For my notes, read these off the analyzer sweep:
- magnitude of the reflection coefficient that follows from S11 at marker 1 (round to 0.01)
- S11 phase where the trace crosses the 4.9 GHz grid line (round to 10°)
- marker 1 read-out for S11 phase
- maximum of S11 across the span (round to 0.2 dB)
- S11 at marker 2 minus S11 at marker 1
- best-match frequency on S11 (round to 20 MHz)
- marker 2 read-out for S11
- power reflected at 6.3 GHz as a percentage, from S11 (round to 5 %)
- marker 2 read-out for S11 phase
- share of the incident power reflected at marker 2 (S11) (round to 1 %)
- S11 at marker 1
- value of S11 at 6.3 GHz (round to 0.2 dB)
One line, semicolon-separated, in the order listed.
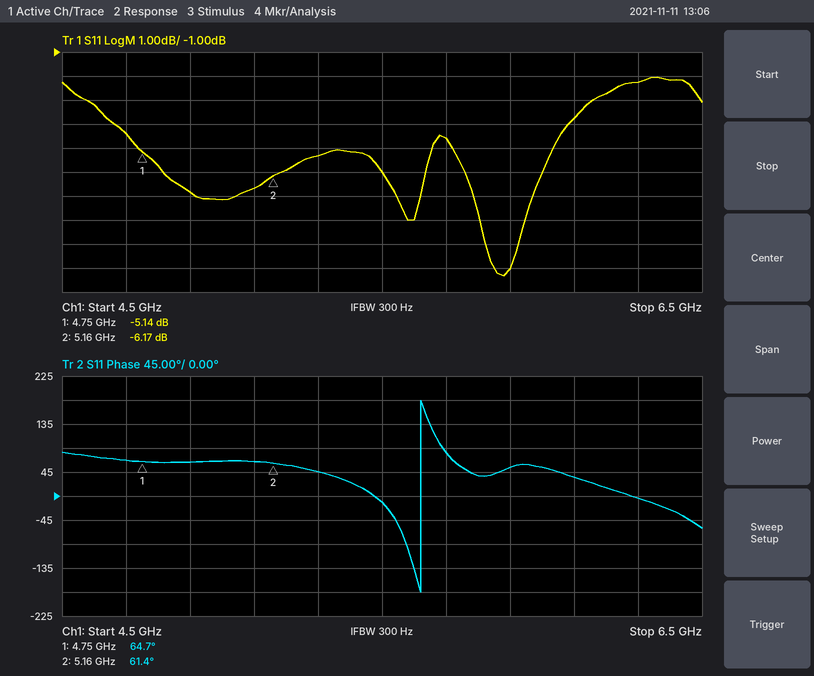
0.55; 60°; 64.7°; -2.0 dB; -1.03 dB; 5.88 GHz; -6.17 dB; 60 %; 61.4°; 24 %; -5.14 dB; -2.2 dB
